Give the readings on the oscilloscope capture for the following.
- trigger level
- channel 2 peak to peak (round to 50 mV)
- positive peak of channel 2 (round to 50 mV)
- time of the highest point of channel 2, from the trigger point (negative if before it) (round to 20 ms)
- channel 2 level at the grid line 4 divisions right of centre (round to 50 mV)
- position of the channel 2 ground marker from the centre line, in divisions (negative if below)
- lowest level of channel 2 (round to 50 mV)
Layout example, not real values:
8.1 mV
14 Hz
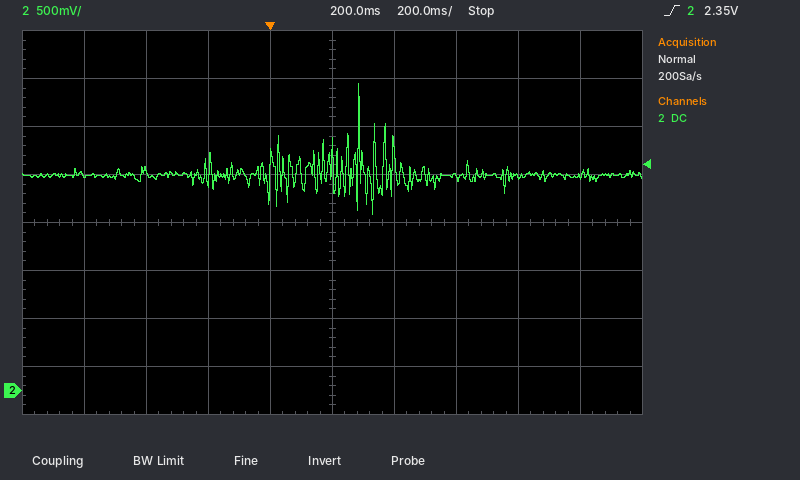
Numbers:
2.35 V
1.35 V
3.20 V
+280 ms
2.25 V
-3.5 div
1.85 V
